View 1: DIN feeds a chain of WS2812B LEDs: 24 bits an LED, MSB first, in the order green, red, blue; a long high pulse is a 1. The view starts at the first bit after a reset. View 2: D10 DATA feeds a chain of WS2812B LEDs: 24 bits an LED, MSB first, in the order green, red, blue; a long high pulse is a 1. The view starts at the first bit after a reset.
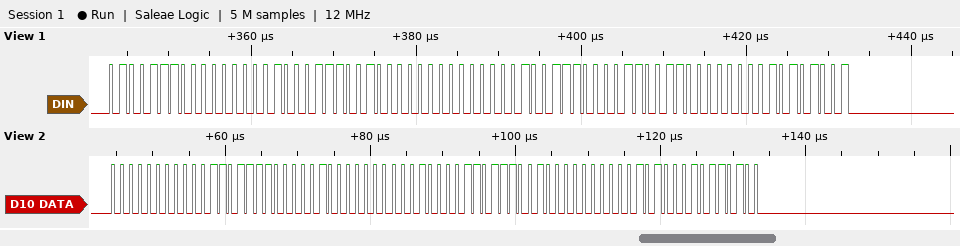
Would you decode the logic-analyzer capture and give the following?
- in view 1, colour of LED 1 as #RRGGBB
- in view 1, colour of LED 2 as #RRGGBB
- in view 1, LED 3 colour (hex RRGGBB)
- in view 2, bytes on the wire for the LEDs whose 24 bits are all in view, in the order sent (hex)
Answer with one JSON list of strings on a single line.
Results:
["#004E8E", "#00409C", "#0033A9", "00 1B C1 00 21 B9 00 28 B4"]
